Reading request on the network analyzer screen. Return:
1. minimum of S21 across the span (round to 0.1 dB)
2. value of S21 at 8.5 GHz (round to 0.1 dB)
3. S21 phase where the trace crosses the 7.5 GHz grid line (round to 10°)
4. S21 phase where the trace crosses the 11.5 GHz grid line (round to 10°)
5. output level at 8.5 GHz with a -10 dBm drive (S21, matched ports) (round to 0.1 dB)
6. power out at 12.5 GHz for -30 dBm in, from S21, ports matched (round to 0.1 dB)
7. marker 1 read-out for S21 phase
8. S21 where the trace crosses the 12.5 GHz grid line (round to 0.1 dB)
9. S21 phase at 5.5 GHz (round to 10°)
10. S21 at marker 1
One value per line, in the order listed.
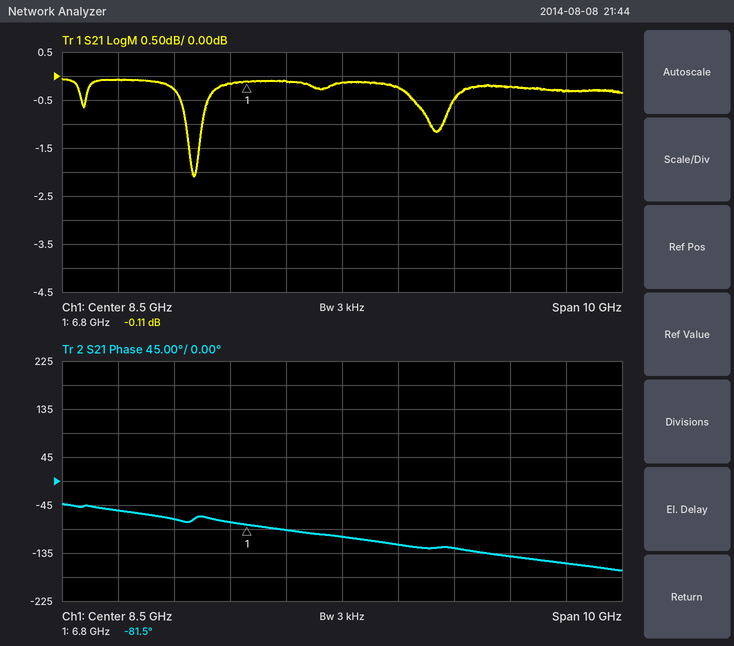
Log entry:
-2.1 dB
-0.1 dB
-90°
-140°
-10.1 dBm
-30.3 dBm
-81.5°
-0.3 dB
-70°
-0.11 dB
